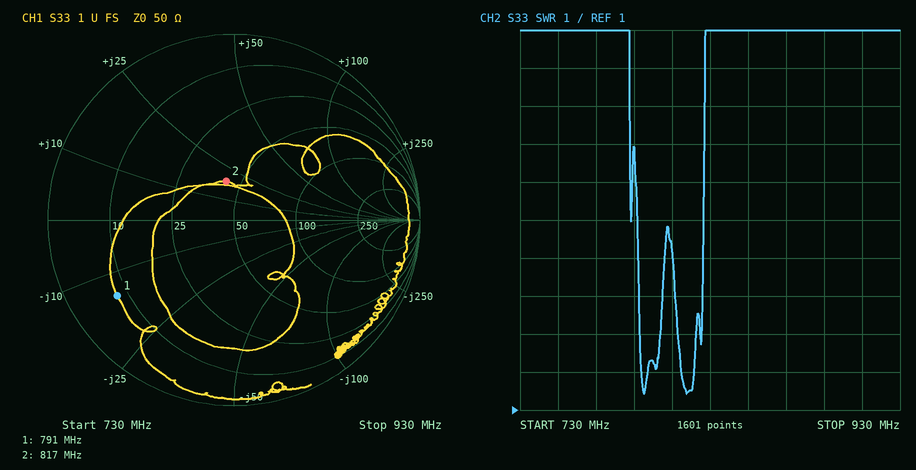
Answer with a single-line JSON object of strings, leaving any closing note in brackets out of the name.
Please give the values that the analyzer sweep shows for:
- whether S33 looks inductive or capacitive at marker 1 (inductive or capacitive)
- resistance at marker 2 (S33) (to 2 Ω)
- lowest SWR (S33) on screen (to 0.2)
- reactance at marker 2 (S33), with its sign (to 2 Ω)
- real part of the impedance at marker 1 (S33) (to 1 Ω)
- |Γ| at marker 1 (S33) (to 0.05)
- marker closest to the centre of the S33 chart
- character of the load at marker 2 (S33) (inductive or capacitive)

{"whether S33 looks inductive or capacitive at marker 1": "capacitive", "resistance at marker 2 (S33)": "42 Ω", "lowest SWR (S33) on screen": "1.4", "reactance at marker 2 (S33), with its sign": "+18 Ω", "real part of the impedance at marker 1 (S33)": "8 Ω", "|Γ| at marker 1 (S33)": "0.75", "marker closest to the centre of the S33 chart": "marker 2", "character of the load at marker 2 (S33)": "inductive"}
